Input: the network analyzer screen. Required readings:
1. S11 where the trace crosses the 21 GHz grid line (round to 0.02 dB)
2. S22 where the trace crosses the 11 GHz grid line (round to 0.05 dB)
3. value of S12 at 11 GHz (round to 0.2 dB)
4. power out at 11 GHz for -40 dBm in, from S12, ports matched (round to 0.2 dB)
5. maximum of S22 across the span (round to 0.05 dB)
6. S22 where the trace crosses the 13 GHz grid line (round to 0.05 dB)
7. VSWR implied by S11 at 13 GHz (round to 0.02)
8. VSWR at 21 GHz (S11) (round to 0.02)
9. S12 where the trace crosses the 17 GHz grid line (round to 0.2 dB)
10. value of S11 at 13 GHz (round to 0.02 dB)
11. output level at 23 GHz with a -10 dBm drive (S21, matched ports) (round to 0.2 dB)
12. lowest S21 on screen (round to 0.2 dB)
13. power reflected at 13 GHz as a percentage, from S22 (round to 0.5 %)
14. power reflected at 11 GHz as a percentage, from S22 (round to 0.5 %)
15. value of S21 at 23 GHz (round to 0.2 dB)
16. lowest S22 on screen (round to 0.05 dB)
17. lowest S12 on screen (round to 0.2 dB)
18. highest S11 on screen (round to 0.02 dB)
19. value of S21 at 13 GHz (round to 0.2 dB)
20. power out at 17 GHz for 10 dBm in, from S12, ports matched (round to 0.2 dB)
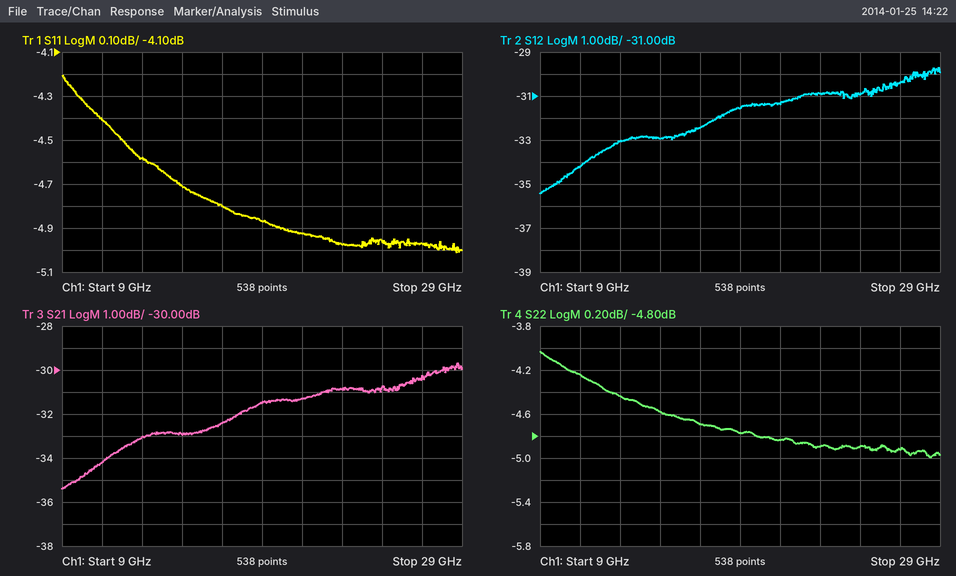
-4.92 dB
-4.25 dB
-34.2 dB
-74.2 dBm
-4.05 dB
-4.45 dB
3.88
3.62
-32.4 dB
-4.58 dB
-40.8 dBm
-35.4 dB
36.0 %
37.5 %
-30.8 dB
-5.00 dB
-35.4 dB
-4.20 dB
-33.0 dB
-22.4 dBm
